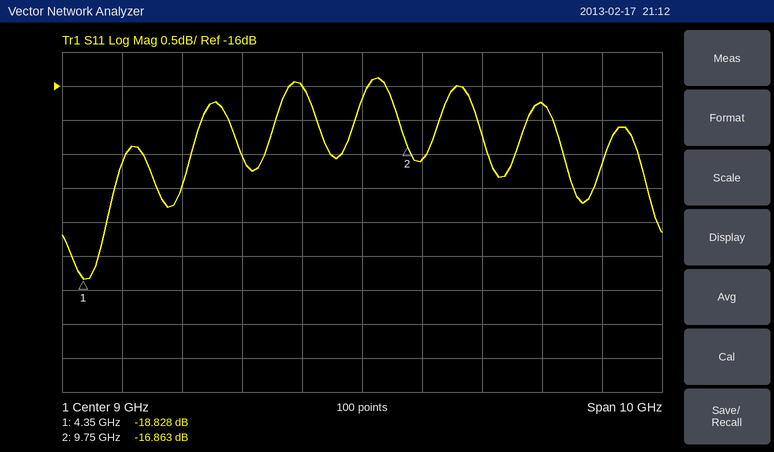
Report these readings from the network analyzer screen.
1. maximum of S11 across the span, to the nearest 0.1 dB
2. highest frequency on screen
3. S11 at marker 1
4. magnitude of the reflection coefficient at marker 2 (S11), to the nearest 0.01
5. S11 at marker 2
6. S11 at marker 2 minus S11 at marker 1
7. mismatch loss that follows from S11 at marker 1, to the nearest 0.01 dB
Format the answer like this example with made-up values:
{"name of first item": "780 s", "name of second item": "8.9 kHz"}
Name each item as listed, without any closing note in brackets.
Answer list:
{"maximum of S11 across the span, to the nearest 0.1 dB": "-15.9 dB", "highest frequency on screen": "14 GHz", "S11 at marker 1": "-18.828 dB", "magnitude of the reflection coefficient at marker 2 (S11), to the nearest 0.01": "0.14", "S11 at marker 2": "-16.863 dB", "S11 at marker 2 minus S11 at marker 1": "1.965 dB", "mismatch loss that follows from S11 at marker 1, to the nearest 0.01 dB": "0.06 dB"}
